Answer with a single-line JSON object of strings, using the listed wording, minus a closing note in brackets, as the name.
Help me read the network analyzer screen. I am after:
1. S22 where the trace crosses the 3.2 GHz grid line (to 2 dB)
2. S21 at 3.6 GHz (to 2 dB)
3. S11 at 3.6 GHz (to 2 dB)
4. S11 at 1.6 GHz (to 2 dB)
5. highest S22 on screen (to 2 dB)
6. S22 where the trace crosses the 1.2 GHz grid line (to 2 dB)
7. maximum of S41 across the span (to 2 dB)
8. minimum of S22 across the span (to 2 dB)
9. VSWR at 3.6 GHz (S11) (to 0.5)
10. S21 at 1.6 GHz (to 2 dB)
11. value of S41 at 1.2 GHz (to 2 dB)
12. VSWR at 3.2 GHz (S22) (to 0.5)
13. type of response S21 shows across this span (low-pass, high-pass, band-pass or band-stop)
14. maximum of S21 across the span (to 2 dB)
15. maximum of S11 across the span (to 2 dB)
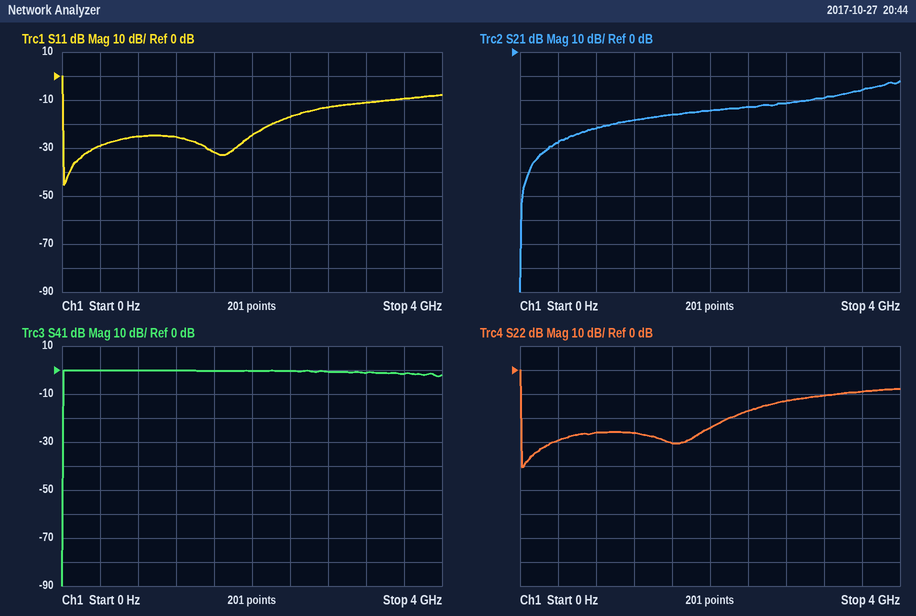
{"S22 where the trace crosses the 3.2 GHz grid line": "-10 dB", "S21 at 3.6 GHz": "-16 dB", "S11 at 3.6 GHz": "-10 dB", "S11 at 1.6 GHz": "-32 dB", "highest S22 on screen": "0 dB", "S22 where the trace crosses the 1.2 GHz grid line": "-26 dB", "maximum of S41 across the span": "0 dB", "minimum of S22 across the span": "-40 dB", "VSWR at 3.6 GHz (S11)": "2.0", "S21 at 1.6 GHz": "-26 dB", "value of S41 at 1.2 GHz": "0 dB", "VSWR at 3.2 GHz (S22)": "2.0", "type of response S21 shows across this span": "high-pass", "maximum of S21 across the span": "-12 dB", "maximum of S11 across the span": "0 dB"}
